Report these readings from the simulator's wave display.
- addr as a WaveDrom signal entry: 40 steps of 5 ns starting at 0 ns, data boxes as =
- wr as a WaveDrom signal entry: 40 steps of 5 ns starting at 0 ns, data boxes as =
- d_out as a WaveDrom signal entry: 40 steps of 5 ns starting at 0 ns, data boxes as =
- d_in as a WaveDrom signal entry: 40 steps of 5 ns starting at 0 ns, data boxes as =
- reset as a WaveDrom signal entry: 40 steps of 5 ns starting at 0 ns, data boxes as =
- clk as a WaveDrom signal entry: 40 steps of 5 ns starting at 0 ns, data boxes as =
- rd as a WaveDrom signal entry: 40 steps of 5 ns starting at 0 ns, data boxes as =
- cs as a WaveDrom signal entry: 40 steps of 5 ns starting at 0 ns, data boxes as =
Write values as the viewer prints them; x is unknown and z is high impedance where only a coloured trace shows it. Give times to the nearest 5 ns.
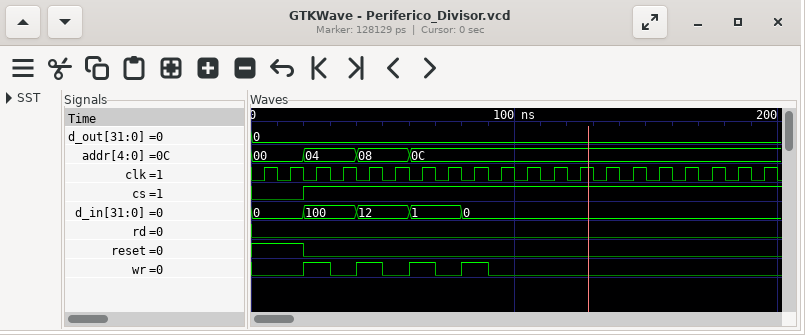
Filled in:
{name: 'addr', wave: '=...=...=...=...........................', data: '00 04 08 0C'}
{name: 'wr', wave: '0...1.0.1.0.1.0.1.0.....................'}
{name: 'd_out', wave: '=.......................................', data: '0'}
{name: 'd_in', wave: '=...=...=...=...=.......................', data: '0 100 12 1 0'}
{name: 'reset', wave: '1...0...................................'}
{name: 'clk', wave: '0101010101010101010101010101010101010101'}
{name: 'rd', wave: '0.......................................'}
{name: 'cs', wave: '0...1...................................'}
